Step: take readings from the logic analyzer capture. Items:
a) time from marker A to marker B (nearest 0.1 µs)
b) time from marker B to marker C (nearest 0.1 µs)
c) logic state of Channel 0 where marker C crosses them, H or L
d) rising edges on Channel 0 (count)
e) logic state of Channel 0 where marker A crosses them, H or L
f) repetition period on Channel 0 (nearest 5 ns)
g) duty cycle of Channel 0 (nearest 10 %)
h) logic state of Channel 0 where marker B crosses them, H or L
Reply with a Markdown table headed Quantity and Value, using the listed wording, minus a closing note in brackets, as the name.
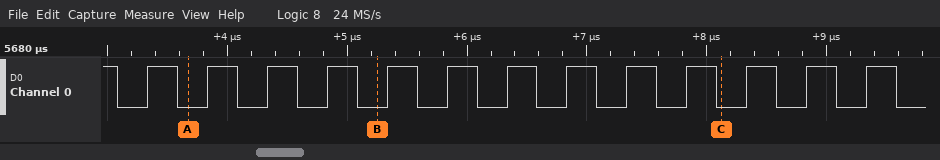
| Quantity | Value |
|---|---|
| time from marker A to marker B | 1.6 µs |
| time from marker B to marker C | 2.9 µs |
| logic state of Channel 0 where marker C crosses them, H or L | Channel 0=L |
| rising edges on Channel 0 | 13 |
| logic state of Channel 0 where marker A crosses them, H or L | Channel 0=L |
| repetition period on Channel 0 | 500 ns |
| duty cycle of Channel 0 | 50 % |
| logic state of Channel 0 where marker B crosses them, H or L | Channel 0=L |
